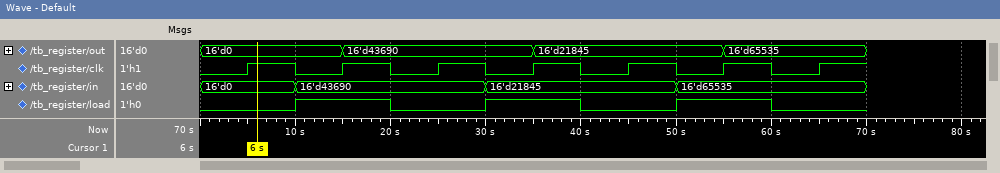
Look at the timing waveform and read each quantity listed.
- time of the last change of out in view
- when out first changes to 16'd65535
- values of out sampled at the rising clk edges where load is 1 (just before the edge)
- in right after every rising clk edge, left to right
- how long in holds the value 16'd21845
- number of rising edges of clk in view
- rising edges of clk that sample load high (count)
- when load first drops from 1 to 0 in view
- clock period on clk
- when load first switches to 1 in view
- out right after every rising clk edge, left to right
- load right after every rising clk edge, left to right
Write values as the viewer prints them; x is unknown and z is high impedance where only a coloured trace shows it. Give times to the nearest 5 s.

55 s
55 s
16'd0, 16'd43690, 16'd21845
16'd0, 16'd43690, 16'd43690, 16'd21845, 16'd21845, 16'd65535, 16'd65535
20 s
7
3
20 s
10 s
10 s
16'd0, 16'd43690, 16'd43690, 16'd21845, 16'd21845, 16'd65535, 16'd65535
0 1 0 1 0 1 0
